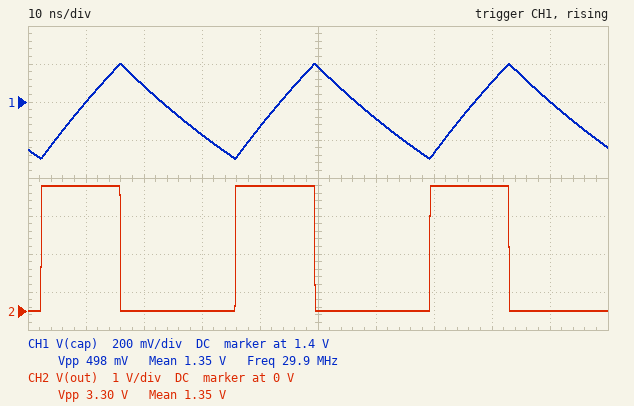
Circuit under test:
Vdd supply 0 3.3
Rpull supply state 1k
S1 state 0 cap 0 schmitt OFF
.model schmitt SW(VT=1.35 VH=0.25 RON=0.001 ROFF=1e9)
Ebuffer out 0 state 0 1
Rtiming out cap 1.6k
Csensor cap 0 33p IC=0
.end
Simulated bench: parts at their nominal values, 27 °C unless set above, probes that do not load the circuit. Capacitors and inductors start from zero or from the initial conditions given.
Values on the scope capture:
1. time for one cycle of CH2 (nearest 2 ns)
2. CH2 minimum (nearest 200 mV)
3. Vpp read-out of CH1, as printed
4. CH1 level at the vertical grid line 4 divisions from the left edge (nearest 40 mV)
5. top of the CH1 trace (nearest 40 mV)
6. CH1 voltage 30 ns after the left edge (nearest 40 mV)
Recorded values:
34 ns
0 V
498 mV
1.28 V
1.60 V
1.24 V
